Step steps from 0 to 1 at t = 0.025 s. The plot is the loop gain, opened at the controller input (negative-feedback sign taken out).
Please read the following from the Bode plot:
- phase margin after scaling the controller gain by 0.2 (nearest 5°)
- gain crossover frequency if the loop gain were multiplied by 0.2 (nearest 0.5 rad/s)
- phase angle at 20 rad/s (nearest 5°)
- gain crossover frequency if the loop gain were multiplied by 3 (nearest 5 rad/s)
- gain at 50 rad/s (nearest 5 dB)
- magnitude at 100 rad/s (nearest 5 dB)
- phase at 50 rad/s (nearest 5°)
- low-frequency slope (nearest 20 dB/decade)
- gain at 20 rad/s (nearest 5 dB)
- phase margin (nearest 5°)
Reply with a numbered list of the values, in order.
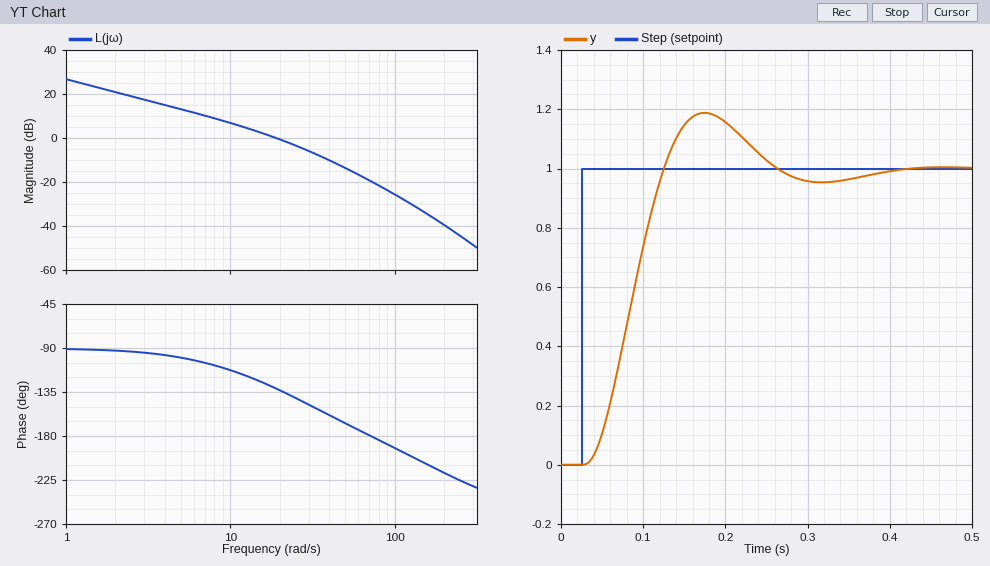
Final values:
1. 80°
2. 4.5 rad/s
3. -135°
4. 40 rad/s
5. -15 dB
6. -25 dB
7. -165°
8. -20 dB/decade
9. 0 dB
10. 50°
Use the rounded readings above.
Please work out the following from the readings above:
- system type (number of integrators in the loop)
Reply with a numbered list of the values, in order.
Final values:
1. 1
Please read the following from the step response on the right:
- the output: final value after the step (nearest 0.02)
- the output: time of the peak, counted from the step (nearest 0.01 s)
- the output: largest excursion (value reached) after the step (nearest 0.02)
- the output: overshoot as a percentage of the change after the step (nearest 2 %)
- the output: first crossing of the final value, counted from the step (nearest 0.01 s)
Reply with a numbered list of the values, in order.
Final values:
1. 1.00
2. 0.15 s
3. 1.18
4. 18 %
5. 0.10 s
